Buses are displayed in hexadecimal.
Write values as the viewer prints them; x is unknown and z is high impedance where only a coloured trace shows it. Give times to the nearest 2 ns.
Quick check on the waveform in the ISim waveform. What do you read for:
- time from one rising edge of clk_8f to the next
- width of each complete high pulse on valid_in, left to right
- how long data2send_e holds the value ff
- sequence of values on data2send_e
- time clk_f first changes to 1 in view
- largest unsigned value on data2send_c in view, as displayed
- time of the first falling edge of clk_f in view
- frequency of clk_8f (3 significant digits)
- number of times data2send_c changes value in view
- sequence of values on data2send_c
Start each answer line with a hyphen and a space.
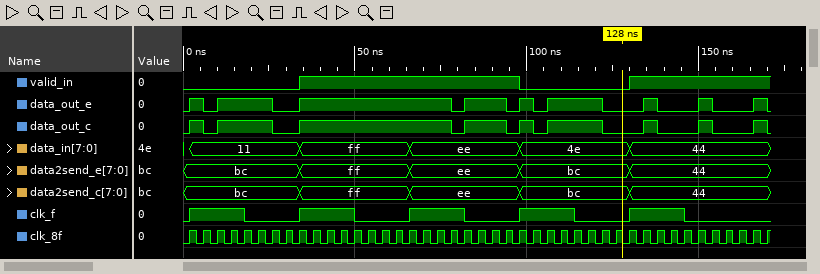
- 4 ns
- 64 ns
- 32 ns
- bc, ff, ee, bc, 44
- 2 ns
- ff
- 18 ns
- 250 MHz
- 4
- bc, ff, ee, bc, 44
